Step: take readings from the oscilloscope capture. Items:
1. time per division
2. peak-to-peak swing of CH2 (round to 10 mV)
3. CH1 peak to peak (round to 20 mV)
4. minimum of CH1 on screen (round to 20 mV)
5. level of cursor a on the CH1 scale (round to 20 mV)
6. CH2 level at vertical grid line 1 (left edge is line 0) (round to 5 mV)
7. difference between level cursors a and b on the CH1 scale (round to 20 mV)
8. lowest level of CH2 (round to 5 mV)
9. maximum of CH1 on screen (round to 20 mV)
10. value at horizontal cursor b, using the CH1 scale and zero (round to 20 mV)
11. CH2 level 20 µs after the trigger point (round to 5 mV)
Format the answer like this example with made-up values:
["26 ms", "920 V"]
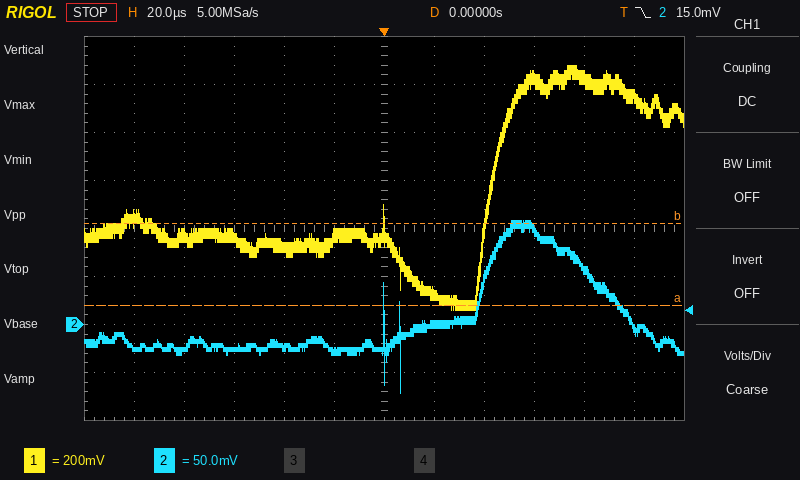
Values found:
["20 µs", "180 mV", "1.02 V", "60 mV", "80 mV", "-25 mV", "340 mV", "-70 mV", "1.08 V", "420 mV", "0 mV"]
